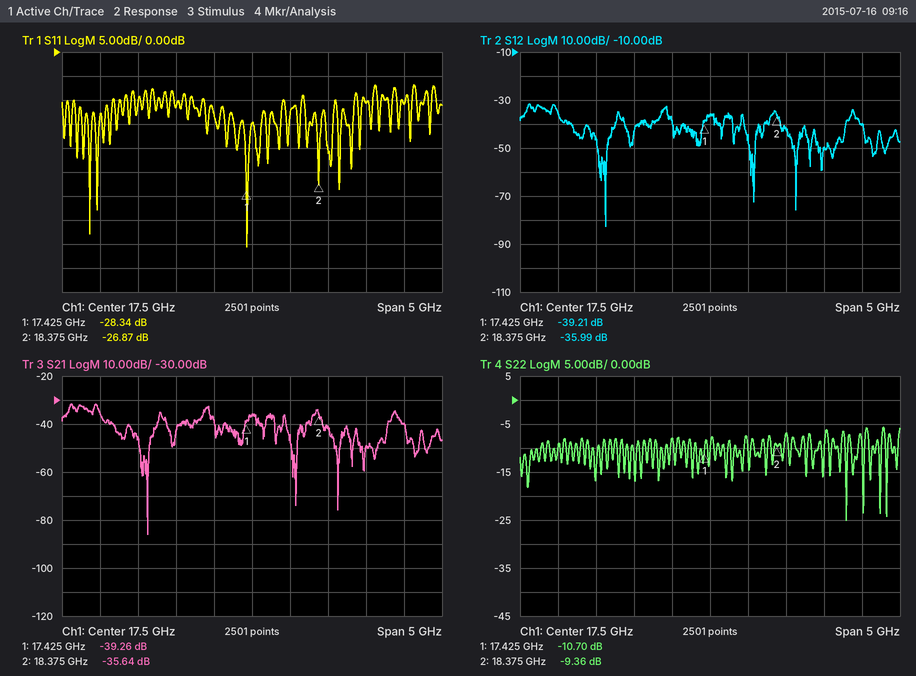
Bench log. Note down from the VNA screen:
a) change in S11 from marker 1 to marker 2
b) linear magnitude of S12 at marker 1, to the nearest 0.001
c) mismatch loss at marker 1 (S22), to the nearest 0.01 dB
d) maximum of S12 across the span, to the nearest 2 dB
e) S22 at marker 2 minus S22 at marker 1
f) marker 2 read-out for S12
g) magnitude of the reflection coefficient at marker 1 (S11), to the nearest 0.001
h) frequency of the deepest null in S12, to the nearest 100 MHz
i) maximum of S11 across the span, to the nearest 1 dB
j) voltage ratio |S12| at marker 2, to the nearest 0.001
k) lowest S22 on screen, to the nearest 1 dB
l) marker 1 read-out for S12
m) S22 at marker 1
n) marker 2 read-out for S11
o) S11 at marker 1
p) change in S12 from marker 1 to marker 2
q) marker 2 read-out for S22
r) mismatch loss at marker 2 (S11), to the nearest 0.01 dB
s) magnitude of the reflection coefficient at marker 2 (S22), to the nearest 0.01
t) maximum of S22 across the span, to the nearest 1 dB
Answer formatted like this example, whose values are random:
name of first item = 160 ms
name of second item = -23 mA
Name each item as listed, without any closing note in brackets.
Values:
change in S11 from marker 1 to marker 2 = 1.47 dB
linear magnitude of S12 at marker 1, to the nearest 0.001 = 0.011
mismatch loss at marker 1 (S22), to the nearest 0.01 dB = 0.39 dB
maximum of S12 across the span, to the nearest 2 dB = -32 dB
S22 at marker 2 minus S22 at marker 1 = 1.34 dB
marker 2 read-out for S12 = -35.99 dB
magnitude of the reflection coefficient at marker 1 (S11), to the nearest 0.001 = 0.038
frequency of the deepest null in S12, to the nearest 100 MHz = 16.1 GHz
maximum of S11 across the span, to the nearest 1 dB = -7 dB
voltage ratio |S12| at marker 2, to the nearest 0.001 = 0.016
lowest S22 on screen, to the nearest 1 dB = -25 dB
marker 1 read-out for S12 = -39.21 dB
S22 at marker 1 = -10.70 dB
marker 2 read-out for S11 = -26.87 dB
S11 at marker 1 = -28.34 dB
change in S12 from marker 1 to marker 2 = 3.22 dB
marker 2 read-out for S22 = -9.36 dB
mismatch loss at marker 2 (S11), to the nearest 0.01 dB = 0.01 dB
magnitude of the reflection coefficient at marker 2 (S22), to the nearest 0.01 = 0.34
maximum of S22 across the span, to the nearest 1 dB = -6 dB
